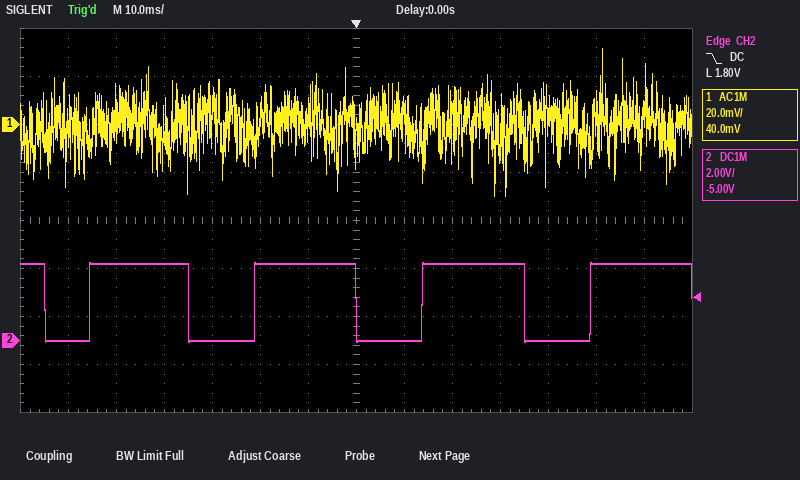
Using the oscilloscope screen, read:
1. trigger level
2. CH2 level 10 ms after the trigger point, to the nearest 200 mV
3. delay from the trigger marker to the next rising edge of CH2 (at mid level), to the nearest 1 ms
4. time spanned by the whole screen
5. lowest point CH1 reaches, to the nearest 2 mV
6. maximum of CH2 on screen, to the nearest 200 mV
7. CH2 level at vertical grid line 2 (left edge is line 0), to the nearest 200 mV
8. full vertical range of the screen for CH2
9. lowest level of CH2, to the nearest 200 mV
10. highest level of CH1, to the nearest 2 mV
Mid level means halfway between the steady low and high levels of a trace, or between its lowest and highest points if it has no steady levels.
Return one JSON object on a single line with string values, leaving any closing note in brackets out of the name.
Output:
{"trigger level": "1.80 V", "CH2 level 10 ms after the trigger point, to the nearest 200 mV": "0.0 V", "delay from the trigger marker to the next rising edge of CH2 (at mid level), to the nearest 1 ms": "14 ms", "time spanned by the whole screen": "140 ms", "lowest point CH1 reaches, to the nearest 2 mV": "-30 mV", "maximum of CH2 on screen, to the nearest 200 mV": "3.2 V", "CH2 level at vertical grid line 2 (left edge is line 0), to the nearest 200 mV": "3.2 V", "full vertical range of the screen for CH2": "16 V", "lowest level of CH2, to the nearest 200 mV": "0.0 V", "highest level of CH1, to the nearest 2 mV": "32 mV"}
